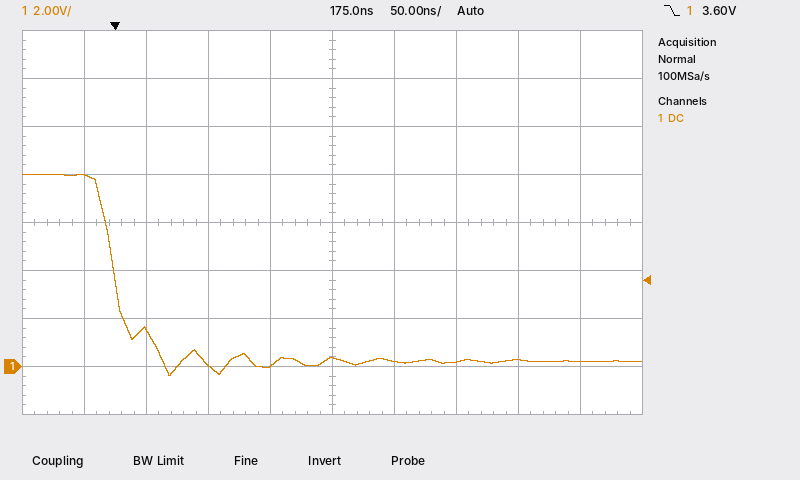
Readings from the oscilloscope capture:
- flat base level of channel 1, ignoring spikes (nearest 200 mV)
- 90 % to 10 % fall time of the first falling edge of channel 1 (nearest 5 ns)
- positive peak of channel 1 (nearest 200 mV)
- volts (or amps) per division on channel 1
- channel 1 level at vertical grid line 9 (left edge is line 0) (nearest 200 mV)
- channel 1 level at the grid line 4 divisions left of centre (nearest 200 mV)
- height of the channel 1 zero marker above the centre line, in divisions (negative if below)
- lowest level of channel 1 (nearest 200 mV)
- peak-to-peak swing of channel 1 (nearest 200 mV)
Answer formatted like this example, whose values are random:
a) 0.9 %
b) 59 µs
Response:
a) 200 mV
b) 45 ns
c) 8.0 V
d) 2 V
e) 200 mV
f) 8.0 V
g) -3.0 div
h) -400 mV
i) 8.4 V
